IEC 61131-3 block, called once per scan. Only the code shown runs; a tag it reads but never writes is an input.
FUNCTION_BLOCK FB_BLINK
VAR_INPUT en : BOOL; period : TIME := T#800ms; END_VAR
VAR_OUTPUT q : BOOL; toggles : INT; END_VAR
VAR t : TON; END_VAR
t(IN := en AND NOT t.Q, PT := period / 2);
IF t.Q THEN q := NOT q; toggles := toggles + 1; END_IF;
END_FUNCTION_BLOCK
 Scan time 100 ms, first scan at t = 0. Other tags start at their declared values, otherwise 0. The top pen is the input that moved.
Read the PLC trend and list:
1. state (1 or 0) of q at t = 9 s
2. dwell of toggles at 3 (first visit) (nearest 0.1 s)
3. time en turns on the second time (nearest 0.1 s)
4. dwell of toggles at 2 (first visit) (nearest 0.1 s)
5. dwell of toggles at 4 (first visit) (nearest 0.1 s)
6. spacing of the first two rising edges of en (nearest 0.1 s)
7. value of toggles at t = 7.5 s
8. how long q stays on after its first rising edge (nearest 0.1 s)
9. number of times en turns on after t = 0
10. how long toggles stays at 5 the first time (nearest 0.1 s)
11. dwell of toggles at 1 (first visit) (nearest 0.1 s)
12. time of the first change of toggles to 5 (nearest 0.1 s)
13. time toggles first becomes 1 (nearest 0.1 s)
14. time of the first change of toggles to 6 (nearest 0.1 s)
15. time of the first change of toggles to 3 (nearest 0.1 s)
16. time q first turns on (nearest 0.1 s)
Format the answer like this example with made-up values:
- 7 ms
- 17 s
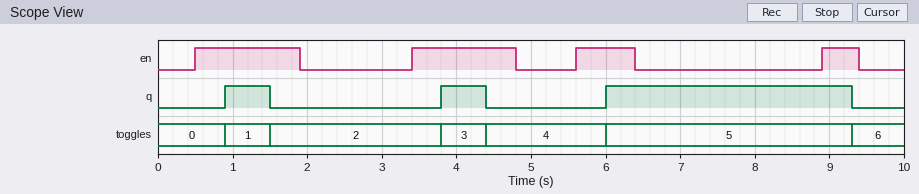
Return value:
- 1
- 0.6 s
- 3.4 s
- 2.3 s
- 1.6 s
- 2.9 s
- 5
- 0.6 s
- 4
- 3.3 s
- 0.6 s
- 6.0 s
- 0.9 s
- 9.3 s
- 3.8 s
- 0.9 s
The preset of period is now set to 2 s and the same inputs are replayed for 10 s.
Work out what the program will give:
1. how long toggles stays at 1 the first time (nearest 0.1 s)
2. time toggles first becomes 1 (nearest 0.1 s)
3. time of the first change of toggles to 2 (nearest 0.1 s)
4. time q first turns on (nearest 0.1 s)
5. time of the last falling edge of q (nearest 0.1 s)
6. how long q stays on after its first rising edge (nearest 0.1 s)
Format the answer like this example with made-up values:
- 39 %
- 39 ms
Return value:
- 2.9 s
- 1.5 s
- 4.4 s
- 1.5 s
- 4.4 s
- 2.9 s
